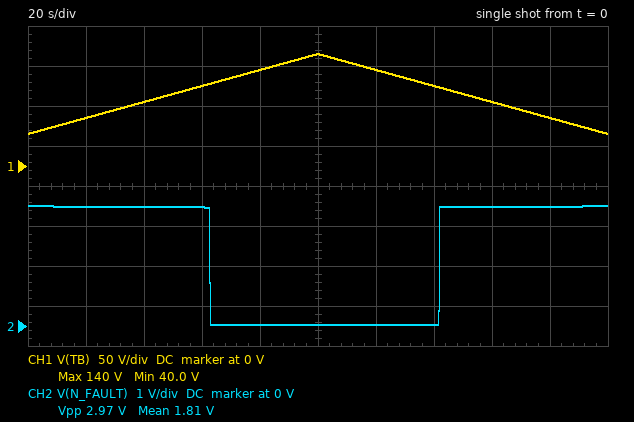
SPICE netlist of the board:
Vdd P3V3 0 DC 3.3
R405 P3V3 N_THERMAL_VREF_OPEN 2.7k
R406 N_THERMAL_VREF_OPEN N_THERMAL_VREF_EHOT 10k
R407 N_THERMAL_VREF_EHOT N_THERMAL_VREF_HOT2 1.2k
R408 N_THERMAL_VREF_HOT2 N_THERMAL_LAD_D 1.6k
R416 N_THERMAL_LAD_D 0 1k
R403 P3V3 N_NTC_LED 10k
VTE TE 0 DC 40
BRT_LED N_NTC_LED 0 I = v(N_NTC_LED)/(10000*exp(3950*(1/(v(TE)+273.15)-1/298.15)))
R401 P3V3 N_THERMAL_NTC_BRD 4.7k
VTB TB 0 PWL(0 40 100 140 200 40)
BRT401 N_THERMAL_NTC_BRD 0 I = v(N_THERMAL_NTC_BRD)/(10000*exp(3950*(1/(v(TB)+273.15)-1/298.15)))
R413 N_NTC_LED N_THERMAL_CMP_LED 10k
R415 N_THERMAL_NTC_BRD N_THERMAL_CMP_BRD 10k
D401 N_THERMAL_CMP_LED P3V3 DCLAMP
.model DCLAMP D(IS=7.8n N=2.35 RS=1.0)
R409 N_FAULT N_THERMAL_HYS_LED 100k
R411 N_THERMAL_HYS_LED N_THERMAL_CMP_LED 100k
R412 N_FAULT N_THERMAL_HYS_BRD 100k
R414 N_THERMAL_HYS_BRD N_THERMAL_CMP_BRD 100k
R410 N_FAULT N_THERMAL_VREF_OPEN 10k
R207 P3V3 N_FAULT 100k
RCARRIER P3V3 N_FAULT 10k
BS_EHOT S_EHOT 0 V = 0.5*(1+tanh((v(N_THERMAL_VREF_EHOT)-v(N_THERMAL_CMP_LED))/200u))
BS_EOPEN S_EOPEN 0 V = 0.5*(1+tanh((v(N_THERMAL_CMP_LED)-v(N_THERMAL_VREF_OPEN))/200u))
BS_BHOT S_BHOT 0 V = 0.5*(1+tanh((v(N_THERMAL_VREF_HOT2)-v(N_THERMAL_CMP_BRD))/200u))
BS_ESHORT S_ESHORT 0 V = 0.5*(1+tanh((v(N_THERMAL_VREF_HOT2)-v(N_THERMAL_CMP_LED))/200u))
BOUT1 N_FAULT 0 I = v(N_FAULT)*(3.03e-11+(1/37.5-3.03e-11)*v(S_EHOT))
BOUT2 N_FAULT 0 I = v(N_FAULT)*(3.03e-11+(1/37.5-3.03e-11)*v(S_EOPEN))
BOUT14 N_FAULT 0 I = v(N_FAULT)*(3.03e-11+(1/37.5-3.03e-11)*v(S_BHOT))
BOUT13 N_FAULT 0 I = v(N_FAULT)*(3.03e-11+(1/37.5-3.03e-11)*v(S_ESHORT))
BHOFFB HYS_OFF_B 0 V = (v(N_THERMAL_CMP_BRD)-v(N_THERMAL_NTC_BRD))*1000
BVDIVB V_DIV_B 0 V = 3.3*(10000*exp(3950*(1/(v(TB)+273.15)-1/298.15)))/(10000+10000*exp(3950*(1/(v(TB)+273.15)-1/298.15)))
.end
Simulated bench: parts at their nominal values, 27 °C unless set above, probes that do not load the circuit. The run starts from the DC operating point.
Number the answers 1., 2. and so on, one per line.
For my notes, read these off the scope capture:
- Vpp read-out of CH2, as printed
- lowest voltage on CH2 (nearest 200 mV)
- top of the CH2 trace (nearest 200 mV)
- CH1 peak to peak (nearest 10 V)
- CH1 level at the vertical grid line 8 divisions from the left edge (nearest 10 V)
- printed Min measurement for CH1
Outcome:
1. 2.97 V
2. 0 V
3. 3.0 V
4. 100 V
5. 80 V
6. 40.0 V
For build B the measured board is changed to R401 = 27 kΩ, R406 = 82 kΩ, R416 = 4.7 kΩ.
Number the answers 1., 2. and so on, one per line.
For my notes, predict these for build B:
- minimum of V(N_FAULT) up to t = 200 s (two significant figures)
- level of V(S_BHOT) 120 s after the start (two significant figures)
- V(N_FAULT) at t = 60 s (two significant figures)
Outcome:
1. 23 mV
2. 1.0 V
3. 3.1 V
